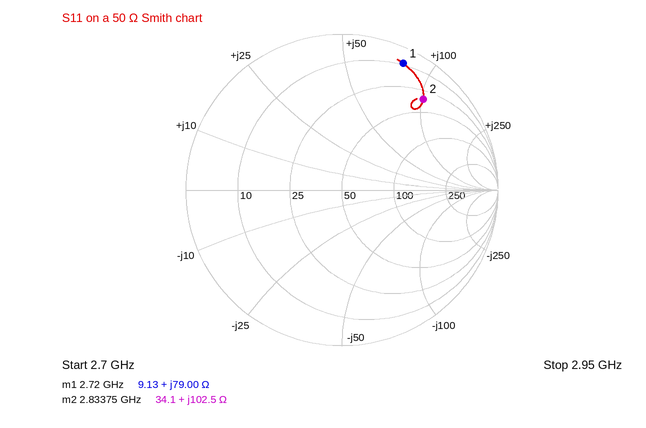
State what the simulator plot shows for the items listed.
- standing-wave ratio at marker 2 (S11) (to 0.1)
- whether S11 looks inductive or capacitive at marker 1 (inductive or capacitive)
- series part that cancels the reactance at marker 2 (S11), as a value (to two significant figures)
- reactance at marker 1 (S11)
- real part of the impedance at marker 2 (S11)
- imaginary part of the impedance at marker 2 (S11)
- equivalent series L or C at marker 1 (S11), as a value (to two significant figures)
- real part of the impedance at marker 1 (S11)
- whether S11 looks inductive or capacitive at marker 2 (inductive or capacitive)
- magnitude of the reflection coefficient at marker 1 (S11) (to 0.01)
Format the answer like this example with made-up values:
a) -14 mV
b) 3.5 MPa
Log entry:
a) 8.2
b) inductive
c) 550 fF
d) +79.00 Ω
e) 34.1 Ω
f) +102.5 Ω
g) 4.6 nH
h) 9.13 Ω
i) inductive
j) 0.90
